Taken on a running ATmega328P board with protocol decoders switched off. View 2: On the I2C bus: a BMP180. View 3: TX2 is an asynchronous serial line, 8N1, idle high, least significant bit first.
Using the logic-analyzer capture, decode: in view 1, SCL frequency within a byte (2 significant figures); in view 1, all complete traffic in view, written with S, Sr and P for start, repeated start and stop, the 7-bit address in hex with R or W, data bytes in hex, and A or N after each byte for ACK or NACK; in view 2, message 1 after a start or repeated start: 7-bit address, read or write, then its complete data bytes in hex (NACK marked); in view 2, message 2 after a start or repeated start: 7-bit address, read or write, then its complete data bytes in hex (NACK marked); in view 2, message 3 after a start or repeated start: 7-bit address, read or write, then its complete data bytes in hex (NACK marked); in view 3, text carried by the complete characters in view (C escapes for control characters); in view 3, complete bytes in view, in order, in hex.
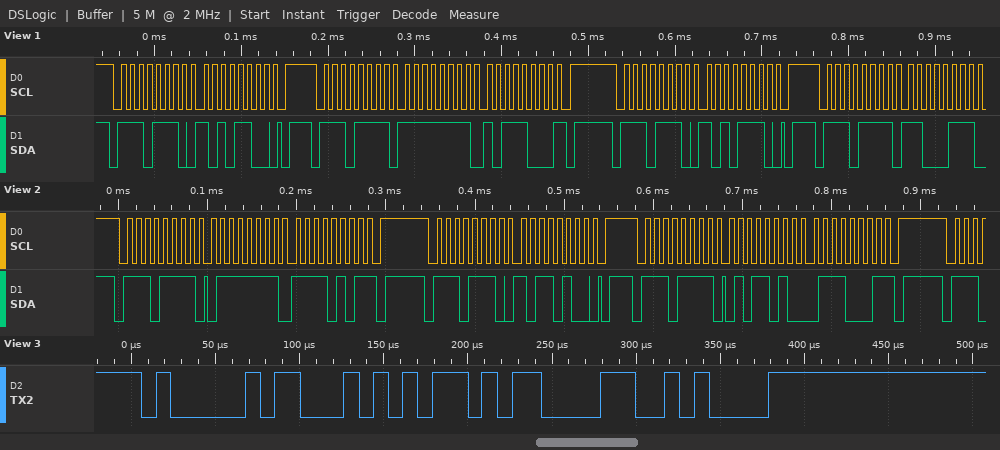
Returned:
100 kHz
S 77W A AC A P S 77R A FF A B8 N P S 77W A AE A P S 77R A C7 A
0x77 read: 7F F5 NACK
0x77 write: B4
0x77 read: 5A 71 NACK
"AT\r\n"
41 54 0D 0A
